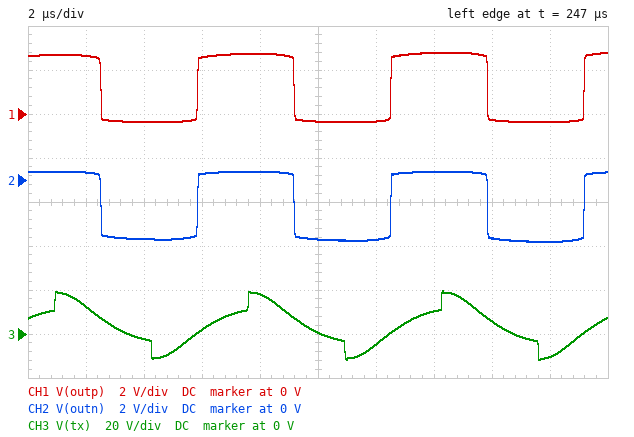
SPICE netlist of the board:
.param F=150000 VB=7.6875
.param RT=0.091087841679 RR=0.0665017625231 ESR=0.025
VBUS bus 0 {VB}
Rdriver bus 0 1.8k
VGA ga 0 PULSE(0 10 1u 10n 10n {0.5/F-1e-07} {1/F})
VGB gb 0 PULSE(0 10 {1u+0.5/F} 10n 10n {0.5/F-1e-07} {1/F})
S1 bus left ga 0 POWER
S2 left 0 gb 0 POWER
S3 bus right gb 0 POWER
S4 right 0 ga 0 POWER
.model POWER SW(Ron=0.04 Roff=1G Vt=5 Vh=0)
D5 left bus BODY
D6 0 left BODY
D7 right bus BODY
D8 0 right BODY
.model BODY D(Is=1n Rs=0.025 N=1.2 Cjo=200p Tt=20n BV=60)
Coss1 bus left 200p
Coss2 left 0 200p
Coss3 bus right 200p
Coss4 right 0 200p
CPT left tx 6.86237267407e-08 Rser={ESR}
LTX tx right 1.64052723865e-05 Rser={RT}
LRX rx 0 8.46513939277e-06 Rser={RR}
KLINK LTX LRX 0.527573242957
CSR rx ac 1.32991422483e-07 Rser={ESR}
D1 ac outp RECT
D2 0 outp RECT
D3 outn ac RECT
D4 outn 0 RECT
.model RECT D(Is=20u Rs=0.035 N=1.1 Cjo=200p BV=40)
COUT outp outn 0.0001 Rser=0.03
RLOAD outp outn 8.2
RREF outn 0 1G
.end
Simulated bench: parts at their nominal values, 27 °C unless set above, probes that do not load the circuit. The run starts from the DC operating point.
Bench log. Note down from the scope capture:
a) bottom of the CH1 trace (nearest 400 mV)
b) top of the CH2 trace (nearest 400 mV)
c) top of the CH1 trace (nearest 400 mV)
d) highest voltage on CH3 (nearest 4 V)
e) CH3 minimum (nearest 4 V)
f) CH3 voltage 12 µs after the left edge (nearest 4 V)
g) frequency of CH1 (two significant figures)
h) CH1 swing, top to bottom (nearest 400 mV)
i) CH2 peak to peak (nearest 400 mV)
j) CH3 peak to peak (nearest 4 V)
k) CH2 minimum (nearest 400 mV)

-400 mV
400 mV
2.8 V
20 V
-12 V
-4 V
150 kHz
3.2 V
3.2 V
32 V
-2.8 V
